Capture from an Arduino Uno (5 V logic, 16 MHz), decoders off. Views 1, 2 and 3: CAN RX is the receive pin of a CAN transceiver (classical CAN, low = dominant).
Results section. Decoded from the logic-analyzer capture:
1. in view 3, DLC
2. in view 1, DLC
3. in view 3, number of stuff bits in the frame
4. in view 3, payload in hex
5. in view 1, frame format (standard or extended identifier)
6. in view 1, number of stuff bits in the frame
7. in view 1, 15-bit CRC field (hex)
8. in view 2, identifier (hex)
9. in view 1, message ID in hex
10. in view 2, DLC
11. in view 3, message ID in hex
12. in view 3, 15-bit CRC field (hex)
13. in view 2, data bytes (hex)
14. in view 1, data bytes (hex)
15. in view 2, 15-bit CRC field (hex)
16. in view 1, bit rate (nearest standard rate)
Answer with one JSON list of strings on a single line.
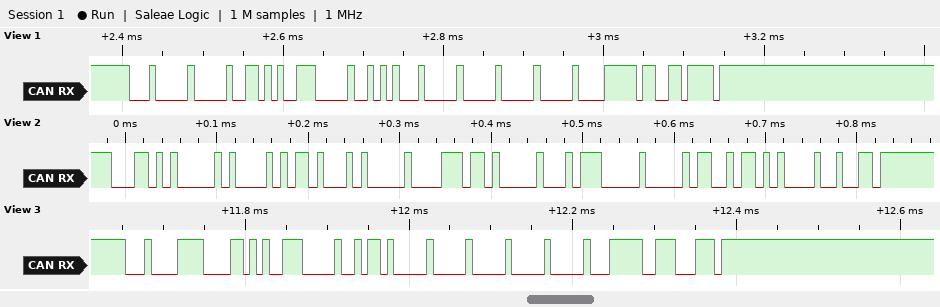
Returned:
["6", "6", "7", "A7 01 68 00 00 00", "standard", "8", "0x7F37", "0x1A8", "0x100", "8", "0x10F", "0x3EE3", "56 8A 00 ED 00 B8 00 CB", "A7 01 51 00 00 00", "0x2849", "125 kbit/s"]
